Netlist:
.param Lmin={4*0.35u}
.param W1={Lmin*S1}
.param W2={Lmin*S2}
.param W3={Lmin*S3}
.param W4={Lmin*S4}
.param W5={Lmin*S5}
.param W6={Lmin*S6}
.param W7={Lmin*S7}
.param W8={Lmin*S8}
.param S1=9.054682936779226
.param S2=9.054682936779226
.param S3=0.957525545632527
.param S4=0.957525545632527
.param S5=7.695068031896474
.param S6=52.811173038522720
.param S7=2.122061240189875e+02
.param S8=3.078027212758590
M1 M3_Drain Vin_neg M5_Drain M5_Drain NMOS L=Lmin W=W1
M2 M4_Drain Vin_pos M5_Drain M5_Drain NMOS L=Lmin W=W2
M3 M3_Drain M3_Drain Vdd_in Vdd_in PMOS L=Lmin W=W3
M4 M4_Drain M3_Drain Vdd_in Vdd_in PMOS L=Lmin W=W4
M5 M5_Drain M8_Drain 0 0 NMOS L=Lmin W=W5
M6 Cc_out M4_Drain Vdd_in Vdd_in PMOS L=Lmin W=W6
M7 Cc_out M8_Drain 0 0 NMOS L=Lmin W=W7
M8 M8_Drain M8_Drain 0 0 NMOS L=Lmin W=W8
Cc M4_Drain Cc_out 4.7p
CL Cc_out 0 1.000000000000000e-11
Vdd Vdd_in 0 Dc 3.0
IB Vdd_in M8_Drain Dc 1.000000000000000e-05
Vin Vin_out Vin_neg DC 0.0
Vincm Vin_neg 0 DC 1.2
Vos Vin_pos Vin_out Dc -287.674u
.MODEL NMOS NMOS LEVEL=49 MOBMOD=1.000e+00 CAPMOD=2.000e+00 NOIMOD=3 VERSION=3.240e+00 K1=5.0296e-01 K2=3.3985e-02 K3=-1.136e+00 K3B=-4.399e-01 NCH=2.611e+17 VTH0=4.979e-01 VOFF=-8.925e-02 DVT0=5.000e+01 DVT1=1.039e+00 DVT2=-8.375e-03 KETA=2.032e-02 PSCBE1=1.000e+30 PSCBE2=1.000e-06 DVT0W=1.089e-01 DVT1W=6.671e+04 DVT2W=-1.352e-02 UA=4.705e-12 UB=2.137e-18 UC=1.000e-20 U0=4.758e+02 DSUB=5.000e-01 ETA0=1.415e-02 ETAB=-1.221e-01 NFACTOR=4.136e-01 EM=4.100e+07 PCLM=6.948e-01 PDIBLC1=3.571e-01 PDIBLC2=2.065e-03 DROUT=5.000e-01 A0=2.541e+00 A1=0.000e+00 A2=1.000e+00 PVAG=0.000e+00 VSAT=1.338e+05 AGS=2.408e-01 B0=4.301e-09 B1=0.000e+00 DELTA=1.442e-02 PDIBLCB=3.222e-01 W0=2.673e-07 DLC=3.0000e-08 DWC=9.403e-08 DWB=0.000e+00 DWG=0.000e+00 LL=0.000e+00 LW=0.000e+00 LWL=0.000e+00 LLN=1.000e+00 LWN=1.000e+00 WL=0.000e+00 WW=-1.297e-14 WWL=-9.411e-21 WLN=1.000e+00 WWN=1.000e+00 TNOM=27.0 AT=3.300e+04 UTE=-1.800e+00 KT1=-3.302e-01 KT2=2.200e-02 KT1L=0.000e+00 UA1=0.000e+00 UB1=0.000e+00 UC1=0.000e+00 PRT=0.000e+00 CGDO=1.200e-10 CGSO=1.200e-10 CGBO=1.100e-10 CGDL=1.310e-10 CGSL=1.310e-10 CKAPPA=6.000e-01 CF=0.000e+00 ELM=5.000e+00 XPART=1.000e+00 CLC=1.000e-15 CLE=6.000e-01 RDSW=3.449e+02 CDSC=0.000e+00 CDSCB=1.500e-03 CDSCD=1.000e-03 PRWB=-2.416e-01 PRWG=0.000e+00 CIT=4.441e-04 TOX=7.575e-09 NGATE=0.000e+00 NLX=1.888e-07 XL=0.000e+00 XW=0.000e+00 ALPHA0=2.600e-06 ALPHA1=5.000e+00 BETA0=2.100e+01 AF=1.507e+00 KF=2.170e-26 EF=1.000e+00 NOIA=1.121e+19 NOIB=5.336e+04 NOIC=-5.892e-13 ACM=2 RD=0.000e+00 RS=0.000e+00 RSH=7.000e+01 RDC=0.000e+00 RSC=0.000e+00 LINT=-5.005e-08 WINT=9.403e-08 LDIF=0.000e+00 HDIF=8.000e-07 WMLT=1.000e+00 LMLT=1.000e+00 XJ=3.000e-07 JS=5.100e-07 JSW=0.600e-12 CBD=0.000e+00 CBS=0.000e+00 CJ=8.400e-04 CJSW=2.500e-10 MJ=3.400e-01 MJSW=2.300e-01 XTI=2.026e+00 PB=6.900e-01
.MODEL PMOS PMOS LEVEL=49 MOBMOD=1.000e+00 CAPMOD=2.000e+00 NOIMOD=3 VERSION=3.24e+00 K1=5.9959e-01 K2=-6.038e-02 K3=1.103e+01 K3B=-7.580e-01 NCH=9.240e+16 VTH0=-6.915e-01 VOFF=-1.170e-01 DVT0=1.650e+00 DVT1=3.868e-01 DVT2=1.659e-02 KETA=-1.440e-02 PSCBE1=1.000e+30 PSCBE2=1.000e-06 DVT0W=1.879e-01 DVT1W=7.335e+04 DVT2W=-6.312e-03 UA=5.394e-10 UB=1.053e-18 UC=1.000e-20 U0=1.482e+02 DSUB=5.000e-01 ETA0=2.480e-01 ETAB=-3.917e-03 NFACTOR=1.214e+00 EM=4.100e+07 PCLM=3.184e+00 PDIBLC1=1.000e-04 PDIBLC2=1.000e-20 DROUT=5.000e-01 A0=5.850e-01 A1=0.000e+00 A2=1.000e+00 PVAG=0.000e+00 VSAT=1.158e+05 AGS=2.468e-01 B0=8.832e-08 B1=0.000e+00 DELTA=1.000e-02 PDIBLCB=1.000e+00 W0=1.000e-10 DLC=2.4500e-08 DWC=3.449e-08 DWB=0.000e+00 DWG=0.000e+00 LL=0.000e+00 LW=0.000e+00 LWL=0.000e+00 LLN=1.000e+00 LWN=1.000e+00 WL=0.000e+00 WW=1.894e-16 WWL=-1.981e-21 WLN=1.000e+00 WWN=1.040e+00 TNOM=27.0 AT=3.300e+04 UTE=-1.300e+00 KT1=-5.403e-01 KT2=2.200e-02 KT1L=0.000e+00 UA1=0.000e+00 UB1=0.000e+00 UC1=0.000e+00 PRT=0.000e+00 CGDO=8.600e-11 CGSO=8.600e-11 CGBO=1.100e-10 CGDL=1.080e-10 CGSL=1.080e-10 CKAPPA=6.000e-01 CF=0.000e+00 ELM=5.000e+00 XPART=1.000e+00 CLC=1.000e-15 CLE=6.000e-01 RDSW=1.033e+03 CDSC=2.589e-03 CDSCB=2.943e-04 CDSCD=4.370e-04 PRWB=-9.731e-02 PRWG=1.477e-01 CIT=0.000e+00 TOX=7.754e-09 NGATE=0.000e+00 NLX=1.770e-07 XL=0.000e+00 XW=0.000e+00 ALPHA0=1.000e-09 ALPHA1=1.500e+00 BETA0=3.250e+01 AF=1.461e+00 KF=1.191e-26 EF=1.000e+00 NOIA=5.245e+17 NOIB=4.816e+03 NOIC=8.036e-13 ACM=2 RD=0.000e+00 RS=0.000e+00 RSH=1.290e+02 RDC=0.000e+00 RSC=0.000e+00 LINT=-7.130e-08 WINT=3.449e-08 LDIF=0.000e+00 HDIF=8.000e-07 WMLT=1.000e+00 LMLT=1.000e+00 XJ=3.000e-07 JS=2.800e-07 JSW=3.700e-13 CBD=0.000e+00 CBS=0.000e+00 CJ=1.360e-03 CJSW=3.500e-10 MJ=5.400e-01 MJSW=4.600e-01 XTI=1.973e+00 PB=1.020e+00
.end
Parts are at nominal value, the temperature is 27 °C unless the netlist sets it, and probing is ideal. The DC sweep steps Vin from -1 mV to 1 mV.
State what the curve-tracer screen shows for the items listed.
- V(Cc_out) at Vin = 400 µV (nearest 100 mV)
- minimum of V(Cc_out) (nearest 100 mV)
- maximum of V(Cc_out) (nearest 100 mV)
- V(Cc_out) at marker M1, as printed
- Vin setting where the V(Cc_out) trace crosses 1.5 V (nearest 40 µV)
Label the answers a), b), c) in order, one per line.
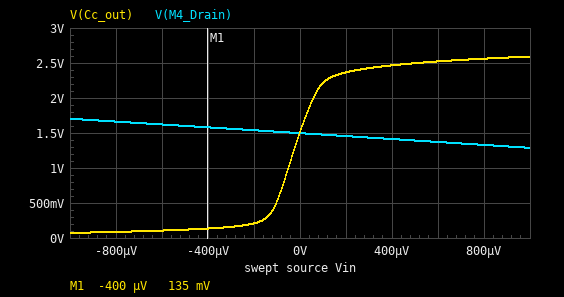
a) 2.5 V
b) 100 mV
c) 2.6 V
d) 135 mV
e) 0 V
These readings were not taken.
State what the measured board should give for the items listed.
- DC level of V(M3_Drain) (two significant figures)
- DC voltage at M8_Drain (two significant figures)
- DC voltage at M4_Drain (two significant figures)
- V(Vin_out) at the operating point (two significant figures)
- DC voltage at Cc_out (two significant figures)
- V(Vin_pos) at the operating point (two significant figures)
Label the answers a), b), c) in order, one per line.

a) 1.4 V
b) 740 mV
c) 1.5 V
d) 1.2 V
e) 1.5 V
f) 1.2 V
